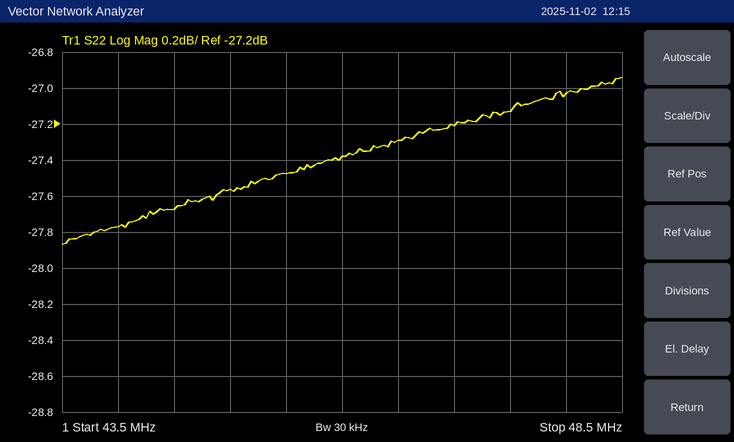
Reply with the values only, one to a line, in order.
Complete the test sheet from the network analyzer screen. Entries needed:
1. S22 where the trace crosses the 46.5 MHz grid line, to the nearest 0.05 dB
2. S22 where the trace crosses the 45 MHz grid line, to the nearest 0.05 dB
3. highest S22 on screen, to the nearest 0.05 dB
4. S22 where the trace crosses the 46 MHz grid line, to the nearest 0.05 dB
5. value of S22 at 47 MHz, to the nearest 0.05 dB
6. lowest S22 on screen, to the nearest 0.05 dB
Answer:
-27.30 dB
-27.55 dB
-26.95 dB
-27.40 dB
-27.20 dB
-27.85 dB
